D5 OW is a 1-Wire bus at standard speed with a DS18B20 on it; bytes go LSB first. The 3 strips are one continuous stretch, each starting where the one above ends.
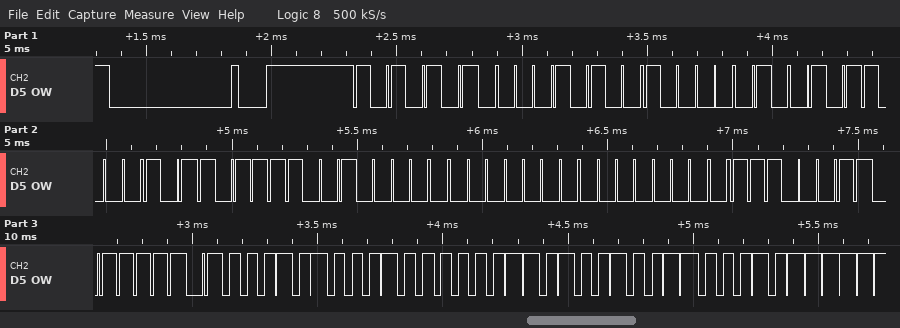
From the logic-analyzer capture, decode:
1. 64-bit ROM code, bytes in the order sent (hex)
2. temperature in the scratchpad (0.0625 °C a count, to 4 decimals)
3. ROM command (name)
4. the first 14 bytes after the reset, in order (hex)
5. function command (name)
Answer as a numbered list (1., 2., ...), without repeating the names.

1. 28 41 1A ED 09 00 00 C7
2. 34.5000 °C
3. Match ROM
4. 55 28 41 1A ED 09 00 00 C7 BE 28 02 4B 46
5. Read Scratchpad
